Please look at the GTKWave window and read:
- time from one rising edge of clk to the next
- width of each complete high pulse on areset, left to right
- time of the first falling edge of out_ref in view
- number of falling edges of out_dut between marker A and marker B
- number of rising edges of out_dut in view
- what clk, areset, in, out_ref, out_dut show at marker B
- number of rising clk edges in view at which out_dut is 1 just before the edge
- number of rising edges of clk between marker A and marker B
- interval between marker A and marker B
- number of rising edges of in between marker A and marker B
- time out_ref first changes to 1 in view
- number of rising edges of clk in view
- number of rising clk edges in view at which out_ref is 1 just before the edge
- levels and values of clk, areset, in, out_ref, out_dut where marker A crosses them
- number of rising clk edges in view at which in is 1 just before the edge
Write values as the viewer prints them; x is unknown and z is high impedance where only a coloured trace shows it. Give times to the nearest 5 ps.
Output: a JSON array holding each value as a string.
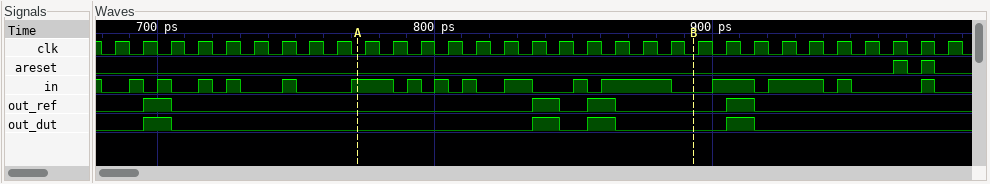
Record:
["10 ps", "5 ps, 5 ps", "705 ps", "2", "4", "clk=0, areset=0, in=0, out_ref=0, out_dut=0", "4", "12", "120 ps", "6", "695 ps", "31", "4", "clk=0, areset=0, in=1, out_ref=0, out_dut=0", "16"]
